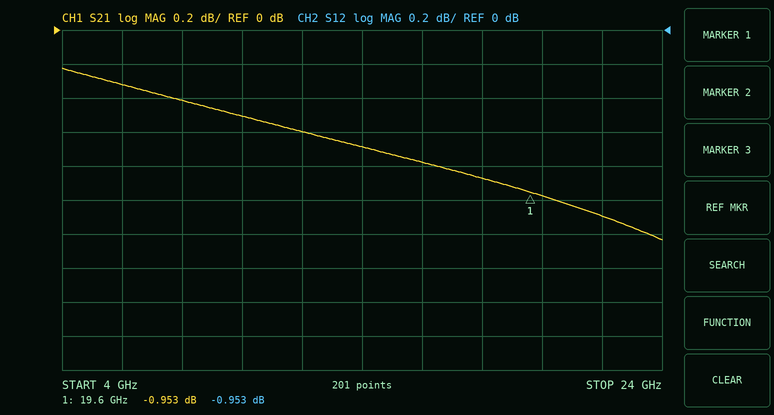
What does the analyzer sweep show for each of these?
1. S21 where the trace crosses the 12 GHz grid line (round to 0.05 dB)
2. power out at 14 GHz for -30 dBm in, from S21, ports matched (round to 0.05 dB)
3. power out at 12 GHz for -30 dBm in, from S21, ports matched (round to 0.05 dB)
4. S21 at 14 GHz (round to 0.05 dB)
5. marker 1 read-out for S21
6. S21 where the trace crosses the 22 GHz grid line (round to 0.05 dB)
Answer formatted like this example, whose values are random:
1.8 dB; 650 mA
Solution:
-0.60 dB; -30.70 dBm; -30.60 dBm; -0.70 dB; -0.953 dB; -1.10 dB
